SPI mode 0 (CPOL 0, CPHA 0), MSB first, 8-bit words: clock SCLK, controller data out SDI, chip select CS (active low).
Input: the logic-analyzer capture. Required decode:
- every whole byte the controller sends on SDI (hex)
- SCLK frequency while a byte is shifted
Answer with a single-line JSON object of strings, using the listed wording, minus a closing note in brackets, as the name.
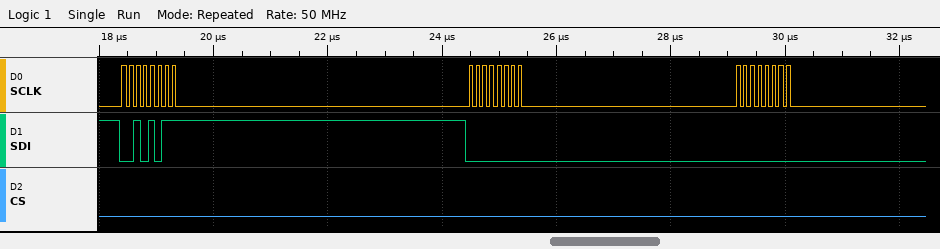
{"every whole byte the controller sends on SDI": "2B 00 00", "SCLK frequency while a byte is shifted": "8 MHz"}
